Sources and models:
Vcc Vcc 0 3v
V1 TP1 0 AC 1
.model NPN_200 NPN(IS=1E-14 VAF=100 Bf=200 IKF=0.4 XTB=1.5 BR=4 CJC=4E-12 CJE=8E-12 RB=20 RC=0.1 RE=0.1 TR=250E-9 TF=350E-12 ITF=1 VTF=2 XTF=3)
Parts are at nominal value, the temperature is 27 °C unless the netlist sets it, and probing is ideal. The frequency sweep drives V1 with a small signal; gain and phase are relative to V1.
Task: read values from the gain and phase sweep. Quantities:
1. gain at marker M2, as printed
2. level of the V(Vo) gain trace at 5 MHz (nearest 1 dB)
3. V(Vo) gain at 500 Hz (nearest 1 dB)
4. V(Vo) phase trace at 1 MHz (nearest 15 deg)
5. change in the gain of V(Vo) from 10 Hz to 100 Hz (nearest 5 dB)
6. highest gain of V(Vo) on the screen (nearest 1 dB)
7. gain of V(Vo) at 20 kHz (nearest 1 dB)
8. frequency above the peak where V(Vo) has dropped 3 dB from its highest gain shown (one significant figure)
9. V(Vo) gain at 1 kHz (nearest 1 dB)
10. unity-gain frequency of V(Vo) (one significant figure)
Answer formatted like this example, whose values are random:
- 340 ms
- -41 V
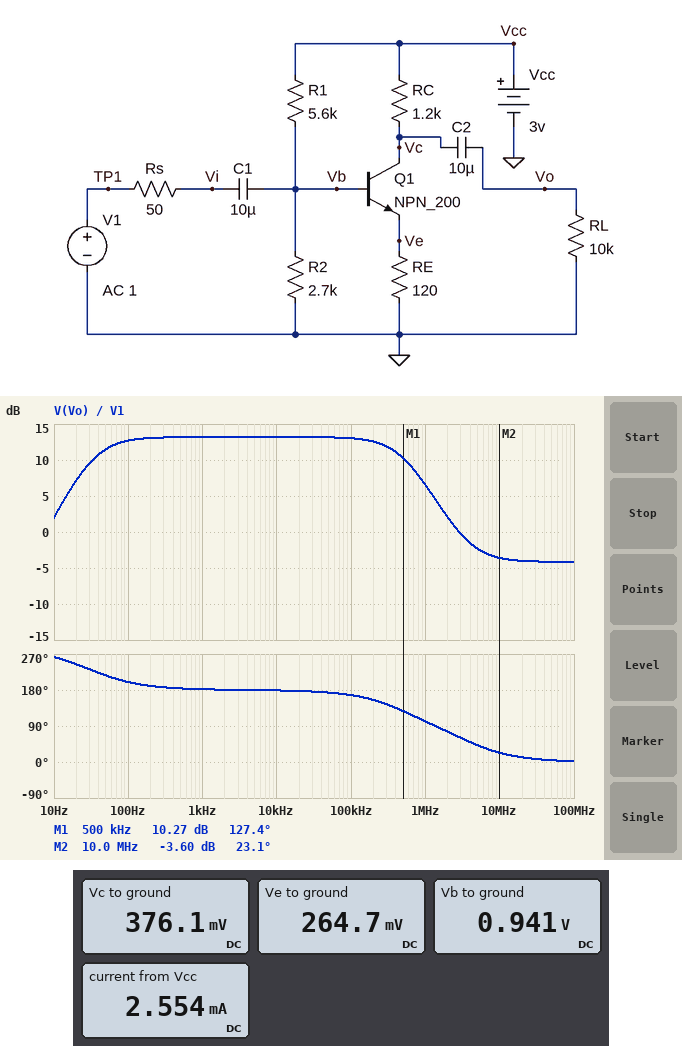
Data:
- -3.60 dB
- -2 dB
- 13 dB
- 105 deg
- 10 dB
- 13 dB
- 13 dB
- 500 kHz
- 13 dB
- 3 MHz
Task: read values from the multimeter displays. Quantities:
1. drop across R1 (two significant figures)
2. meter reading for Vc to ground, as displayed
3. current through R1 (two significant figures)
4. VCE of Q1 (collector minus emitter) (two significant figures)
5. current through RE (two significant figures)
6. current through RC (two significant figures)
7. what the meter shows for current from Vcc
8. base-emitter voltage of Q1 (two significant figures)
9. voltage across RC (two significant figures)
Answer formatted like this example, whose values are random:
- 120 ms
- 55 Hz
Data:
- 2.1 V
- 376.1 mV
- 370 µA
- 110 mV
- 2.2 mA
- 2.2 mA
- 2.554 mA
- 680 mV
- 2.6 V
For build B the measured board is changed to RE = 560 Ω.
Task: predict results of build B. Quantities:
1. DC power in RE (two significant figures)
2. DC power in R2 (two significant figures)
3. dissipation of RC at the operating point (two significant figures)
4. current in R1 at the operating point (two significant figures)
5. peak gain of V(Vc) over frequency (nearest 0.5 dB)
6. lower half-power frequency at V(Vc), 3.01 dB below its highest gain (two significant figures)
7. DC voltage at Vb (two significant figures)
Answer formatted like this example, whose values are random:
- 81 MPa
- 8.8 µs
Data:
- 190 µW
- 350 µW
- 410 µW
- 360 µA
- 4.5 dB
- 8.6 Hz
- 970 mV
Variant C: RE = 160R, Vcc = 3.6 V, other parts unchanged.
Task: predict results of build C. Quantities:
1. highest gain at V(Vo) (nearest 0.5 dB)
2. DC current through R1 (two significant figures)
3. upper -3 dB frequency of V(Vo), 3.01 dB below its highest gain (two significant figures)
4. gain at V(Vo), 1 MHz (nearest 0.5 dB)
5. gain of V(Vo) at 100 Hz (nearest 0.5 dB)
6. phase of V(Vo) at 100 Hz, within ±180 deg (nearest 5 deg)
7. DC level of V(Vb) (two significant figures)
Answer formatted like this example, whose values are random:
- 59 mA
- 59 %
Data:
- 5.0 dB
- 450 µA
- 340 kHz
- -2.0 dB
- 4.0 dB
- -155 deg
- 1.1 V
